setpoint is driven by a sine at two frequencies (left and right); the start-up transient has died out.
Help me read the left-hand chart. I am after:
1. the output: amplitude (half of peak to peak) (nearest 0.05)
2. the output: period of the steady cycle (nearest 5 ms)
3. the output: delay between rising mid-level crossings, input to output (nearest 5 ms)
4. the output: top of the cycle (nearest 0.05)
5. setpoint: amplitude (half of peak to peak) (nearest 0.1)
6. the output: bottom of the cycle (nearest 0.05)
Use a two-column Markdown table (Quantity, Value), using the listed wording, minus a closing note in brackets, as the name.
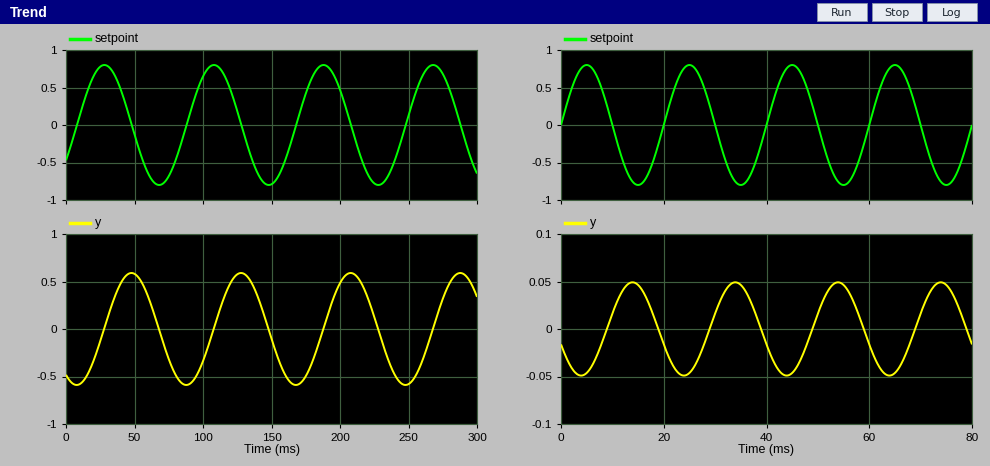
| Quantity | Value |
|---|---|
| the output: amplitude (half of peak to peak) | 0.60 |
| the output: period of the steady cycle | 80 ms |
| the output: delay between rising mid-level crossings, input to output | 20 ms |
| the output: top of the cycle | 0.60 |
| setpoint: amplitude (half of peak to peak) | 0.8 |
| the output: bottom of the cycle | -0.60 |
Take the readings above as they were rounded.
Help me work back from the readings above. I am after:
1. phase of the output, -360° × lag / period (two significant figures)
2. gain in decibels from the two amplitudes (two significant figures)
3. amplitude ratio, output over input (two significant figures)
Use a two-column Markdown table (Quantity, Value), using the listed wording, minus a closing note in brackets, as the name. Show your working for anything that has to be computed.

| Quantity | Value |
|---|---|
| phase of the output, -360° × lag / period | -360 × 20 / 80 = -90° |
| gain in decibels from the two amplitudes | 20 log10(0.6 / 0.8) = -2.5 dB |
| amplitude ratio, output over input | 0.6 / 0.8 = 0.75 |
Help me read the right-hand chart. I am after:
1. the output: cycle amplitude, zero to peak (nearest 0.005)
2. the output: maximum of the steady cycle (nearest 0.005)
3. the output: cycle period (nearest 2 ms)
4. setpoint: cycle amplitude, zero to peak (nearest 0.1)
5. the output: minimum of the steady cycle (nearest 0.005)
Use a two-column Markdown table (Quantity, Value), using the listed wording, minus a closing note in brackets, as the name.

| Quantity | Value |
|---|---|
| the output: cycle amplitude, zero to peak | 0.050 |
| the output: maximum of the steady cycle | 0.050 |
| the output: cycle period | 20 ms |
| setpoint: cycle amplitude, zero to peak | 0.8 |
| the output: minimum of the steady cycle | -0.050 |
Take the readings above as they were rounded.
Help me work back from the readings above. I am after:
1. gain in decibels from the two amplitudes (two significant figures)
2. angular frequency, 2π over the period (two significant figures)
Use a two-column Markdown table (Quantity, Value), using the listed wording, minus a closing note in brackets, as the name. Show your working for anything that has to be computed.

| Quantity | Value |
|---|---|
| gain in decibels from the two amplitudes | 20 log10(0.05 / 0.8) = -24 dB |
| angular frequency, 2π over the period | 2π / 20 = 0.31 rad/ms |
